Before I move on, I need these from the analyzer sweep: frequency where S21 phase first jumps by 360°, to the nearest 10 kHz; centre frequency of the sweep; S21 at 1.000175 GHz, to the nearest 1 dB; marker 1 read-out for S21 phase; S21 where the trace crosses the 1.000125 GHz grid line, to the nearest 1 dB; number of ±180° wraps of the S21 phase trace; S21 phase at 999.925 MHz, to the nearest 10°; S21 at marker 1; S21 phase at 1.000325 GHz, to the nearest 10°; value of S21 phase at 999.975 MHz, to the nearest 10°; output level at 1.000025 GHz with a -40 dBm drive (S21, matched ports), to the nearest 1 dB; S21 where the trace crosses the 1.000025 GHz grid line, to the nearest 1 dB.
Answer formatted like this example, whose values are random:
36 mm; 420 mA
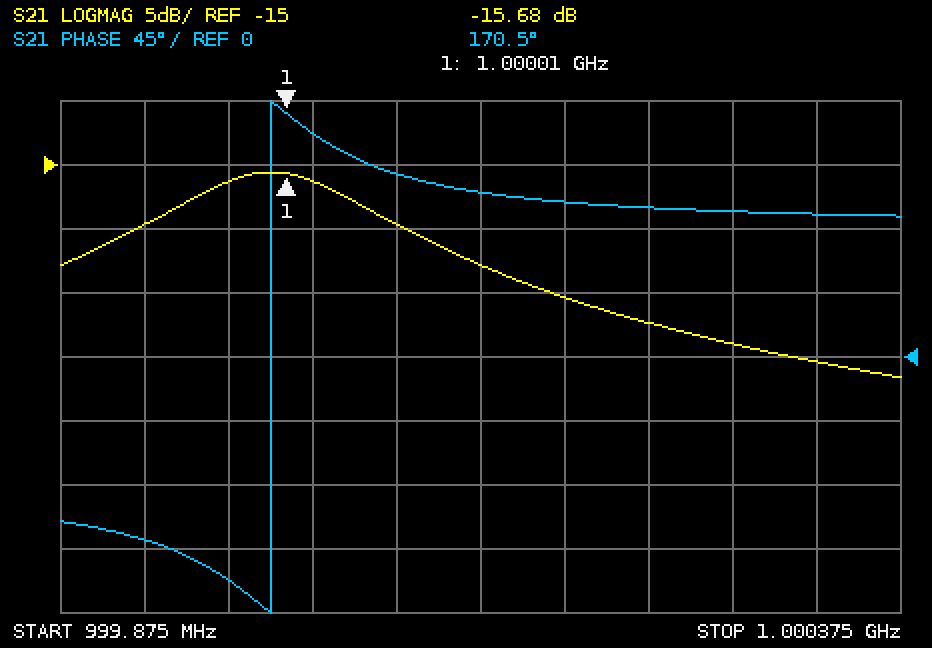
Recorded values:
1.00000 GHz; 1.000125 GHz; -25 dB; 170.5°; -23 dB; 1; -130°; -15.68 dB; 100°; -160°; -56 dBm; -16 dB
